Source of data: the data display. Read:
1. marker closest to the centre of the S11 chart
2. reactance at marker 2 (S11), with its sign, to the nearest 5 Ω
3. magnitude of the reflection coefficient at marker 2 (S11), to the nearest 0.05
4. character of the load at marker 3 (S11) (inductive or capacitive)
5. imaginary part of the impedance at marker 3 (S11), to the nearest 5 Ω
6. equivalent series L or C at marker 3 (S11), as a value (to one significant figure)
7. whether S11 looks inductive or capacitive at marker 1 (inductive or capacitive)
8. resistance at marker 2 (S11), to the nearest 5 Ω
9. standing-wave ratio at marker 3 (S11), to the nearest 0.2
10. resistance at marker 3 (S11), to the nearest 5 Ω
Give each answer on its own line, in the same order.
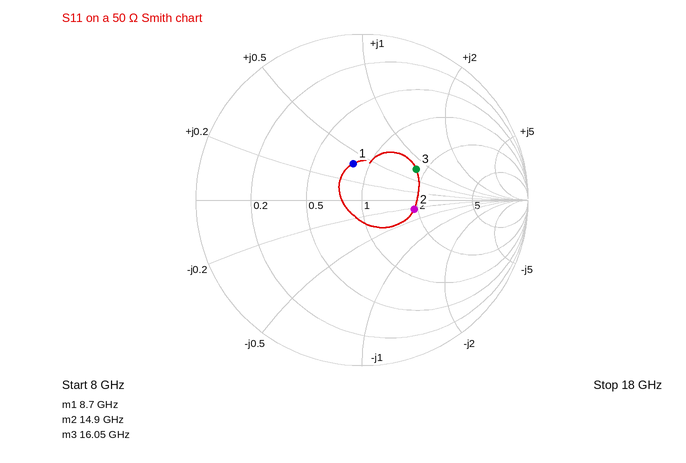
marker 1
-10 Ω
0.30
inductive
+40 Ω
400 pH
inductive
95 Ω
2.2
90 Ω
